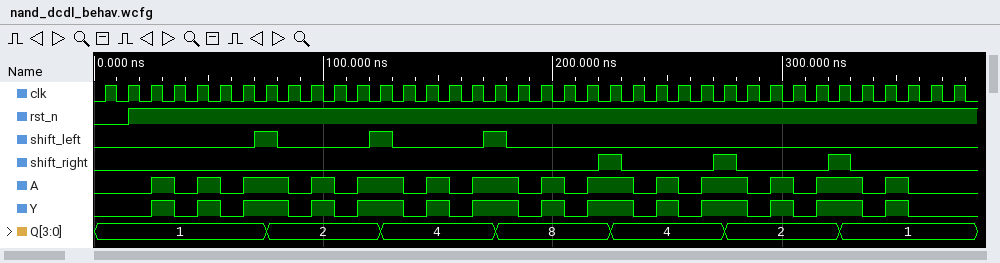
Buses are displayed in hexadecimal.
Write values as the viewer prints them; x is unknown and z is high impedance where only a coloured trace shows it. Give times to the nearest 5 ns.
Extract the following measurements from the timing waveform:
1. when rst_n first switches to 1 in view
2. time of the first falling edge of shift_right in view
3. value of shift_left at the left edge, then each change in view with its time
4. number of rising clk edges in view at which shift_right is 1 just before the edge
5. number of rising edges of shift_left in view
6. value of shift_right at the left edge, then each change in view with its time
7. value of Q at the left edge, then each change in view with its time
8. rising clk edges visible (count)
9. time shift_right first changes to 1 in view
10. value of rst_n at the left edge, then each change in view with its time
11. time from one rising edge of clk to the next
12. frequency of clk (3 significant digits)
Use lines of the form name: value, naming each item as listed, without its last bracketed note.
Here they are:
when rst_n first switches to 1 in view: 15 ns
time of the first falling edge of shift_right in view: 230 ns
value of shift_left at the left edge, then each change in view with its time: 0, 1 at 70 ns, 0 at 80 ns, 1 at 120 ns, 0 at 130 ns, 1 at 170 ns, 0 at 180 ns
number of rising clk edges in view at which shift_right is 1 just before the edge: 3
number of rising edges of shift_left in view: 3
value of shift_right at the left edge, then each change in view with its time: 0, 1 at 220 ns, 0 at 230 ns, 1 at 270 ns, 0 at 280 ns, 1 at 320 ns, 0 at 330 ns
value of Q at the left edge, then each change in view with its time: 1, 2 at 75 ns, 4 at 125 ns, 8 at 175 ns, 4 at 225 ns, 2 at 275 ns, 1 at 325 ns
rising clk edges visible: 38
time shift_right first changes to 1 in view: 220 ns
value of rst_n at the left edge, then each change in view with its time: 0, 1 at 15 ns
time from one rising edge of clk to the next: 10 ns
frequency of clk: 100 MHz
